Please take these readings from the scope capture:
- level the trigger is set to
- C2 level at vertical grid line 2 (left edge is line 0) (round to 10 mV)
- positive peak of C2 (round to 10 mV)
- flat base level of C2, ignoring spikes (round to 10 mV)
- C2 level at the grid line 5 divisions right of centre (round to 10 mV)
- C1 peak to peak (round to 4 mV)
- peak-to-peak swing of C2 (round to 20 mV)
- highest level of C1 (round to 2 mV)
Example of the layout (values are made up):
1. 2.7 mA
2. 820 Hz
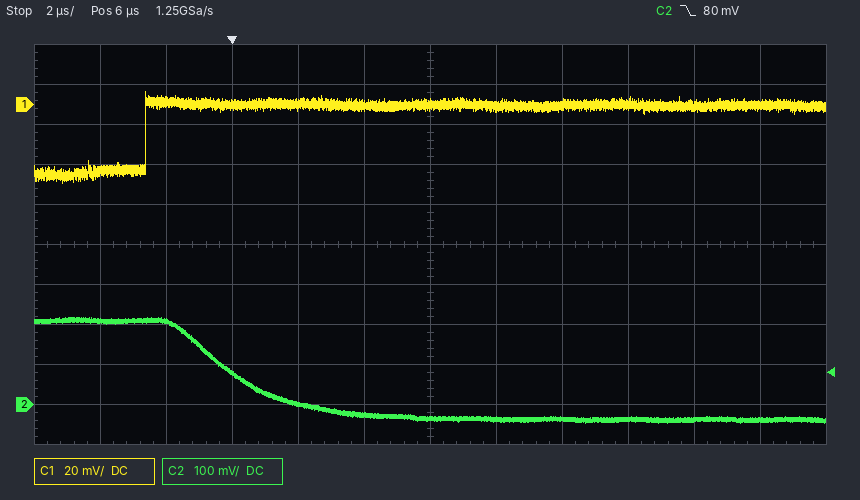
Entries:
1. 80 mV
2. 210 mV
3. 220 mV
4. -40 mV
5. -40 mV
6. 44 mV
7. 260 mV
8. 6 mV
